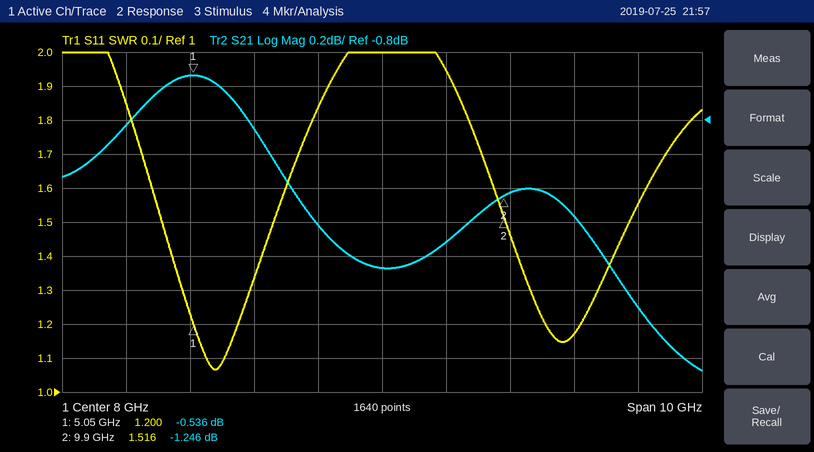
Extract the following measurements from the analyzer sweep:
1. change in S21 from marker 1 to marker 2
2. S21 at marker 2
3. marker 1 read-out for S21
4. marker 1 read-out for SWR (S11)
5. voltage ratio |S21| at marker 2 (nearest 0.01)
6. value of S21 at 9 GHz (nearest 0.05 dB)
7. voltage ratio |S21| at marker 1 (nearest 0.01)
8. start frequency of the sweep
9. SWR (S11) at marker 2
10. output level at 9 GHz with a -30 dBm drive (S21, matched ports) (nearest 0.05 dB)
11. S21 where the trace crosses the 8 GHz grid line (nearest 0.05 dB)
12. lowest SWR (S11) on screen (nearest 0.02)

-0.710 dB
-1.246 dB
-0.536 dB
1.200
0.87
-1.50 dB
0.94
3 GHz
1.516
-31.50 dBm
-1.65 dB
1.06
